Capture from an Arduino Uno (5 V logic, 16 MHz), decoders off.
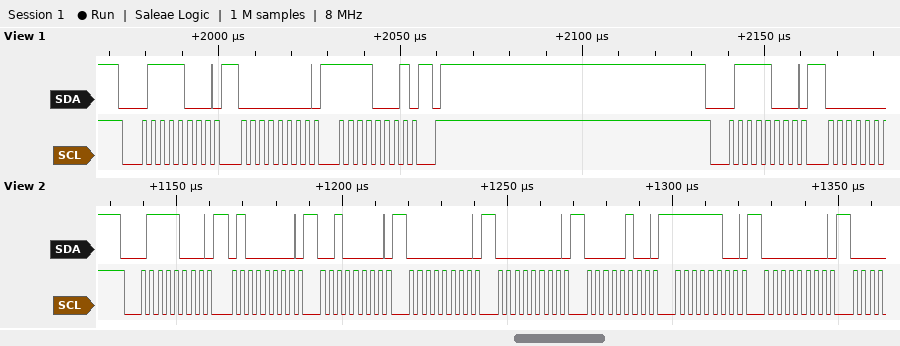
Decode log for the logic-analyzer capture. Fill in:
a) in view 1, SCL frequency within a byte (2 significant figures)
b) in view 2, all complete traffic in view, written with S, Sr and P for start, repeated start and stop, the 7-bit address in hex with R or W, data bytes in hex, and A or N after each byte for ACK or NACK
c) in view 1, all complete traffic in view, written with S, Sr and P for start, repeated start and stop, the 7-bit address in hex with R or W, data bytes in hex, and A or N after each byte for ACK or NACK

400 kHz
S 3CW A 40 A 20 A 00 A 00 A 04 A FC A 00 A
S 3CW A 00 A F1 A P S 3CW A
